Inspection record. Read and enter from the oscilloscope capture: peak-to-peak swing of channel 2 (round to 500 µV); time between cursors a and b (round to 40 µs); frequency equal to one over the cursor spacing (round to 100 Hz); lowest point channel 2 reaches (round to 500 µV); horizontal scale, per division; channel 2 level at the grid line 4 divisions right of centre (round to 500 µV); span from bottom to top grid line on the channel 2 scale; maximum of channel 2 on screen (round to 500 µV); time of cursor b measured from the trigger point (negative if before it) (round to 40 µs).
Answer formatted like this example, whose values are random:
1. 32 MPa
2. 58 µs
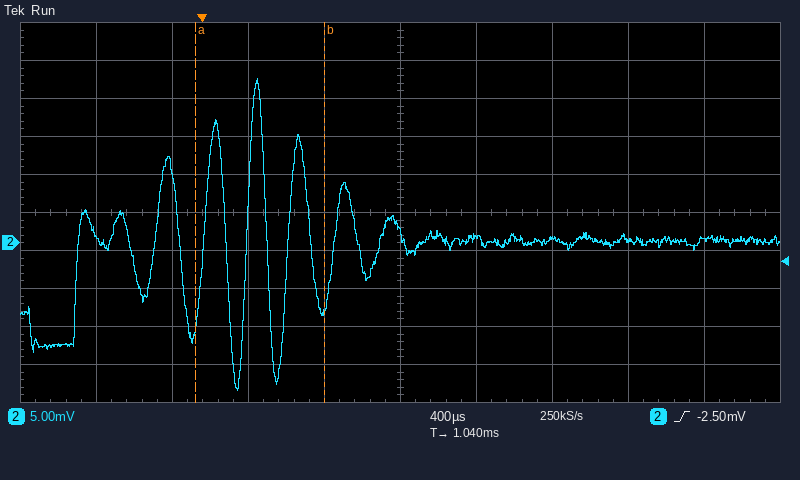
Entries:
1. 41.0 mV
2. 680 µs
3. 1.5 kHz
4. -19.5 mV
5. 400 µs
6. 500 µV
7. 50 mV
8. 21.5 mV
9. +640 µs
